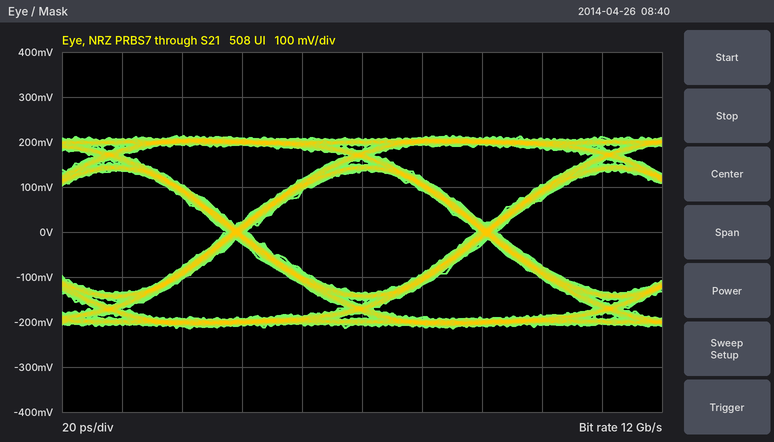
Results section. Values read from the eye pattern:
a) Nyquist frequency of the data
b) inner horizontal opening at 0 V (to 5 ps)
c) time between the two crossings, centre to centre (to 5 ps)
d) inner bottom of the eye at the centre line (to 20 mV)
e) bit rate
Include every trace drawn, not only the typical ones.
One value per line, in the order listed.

6 GHz
75 ps
85 ps
-140 mV
12 Gb/s
